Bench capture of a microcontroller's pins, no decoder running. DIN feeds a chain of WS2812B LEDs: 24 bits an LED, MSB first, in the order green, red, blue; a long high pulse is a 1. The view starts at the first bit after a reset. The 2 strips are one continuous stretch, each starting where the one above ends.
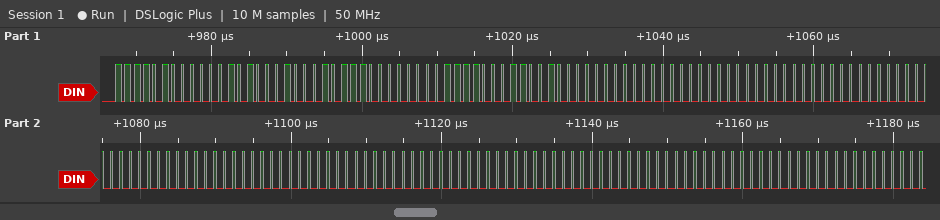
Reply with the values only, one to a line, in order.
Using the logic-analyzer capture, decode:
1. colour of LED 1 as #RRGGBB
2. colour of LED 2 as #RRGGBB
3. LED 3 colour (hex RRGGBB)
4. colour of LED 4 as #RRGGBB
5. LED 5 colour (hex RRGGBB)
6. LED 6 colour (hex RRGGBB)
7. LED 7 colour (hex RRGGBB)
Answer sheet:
#0AF422
#1EE032
#000000
#000000
#000000
#000000
#000000
